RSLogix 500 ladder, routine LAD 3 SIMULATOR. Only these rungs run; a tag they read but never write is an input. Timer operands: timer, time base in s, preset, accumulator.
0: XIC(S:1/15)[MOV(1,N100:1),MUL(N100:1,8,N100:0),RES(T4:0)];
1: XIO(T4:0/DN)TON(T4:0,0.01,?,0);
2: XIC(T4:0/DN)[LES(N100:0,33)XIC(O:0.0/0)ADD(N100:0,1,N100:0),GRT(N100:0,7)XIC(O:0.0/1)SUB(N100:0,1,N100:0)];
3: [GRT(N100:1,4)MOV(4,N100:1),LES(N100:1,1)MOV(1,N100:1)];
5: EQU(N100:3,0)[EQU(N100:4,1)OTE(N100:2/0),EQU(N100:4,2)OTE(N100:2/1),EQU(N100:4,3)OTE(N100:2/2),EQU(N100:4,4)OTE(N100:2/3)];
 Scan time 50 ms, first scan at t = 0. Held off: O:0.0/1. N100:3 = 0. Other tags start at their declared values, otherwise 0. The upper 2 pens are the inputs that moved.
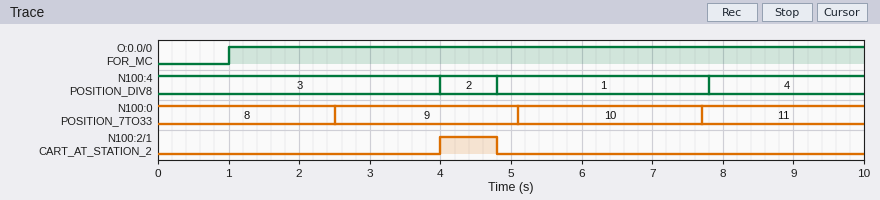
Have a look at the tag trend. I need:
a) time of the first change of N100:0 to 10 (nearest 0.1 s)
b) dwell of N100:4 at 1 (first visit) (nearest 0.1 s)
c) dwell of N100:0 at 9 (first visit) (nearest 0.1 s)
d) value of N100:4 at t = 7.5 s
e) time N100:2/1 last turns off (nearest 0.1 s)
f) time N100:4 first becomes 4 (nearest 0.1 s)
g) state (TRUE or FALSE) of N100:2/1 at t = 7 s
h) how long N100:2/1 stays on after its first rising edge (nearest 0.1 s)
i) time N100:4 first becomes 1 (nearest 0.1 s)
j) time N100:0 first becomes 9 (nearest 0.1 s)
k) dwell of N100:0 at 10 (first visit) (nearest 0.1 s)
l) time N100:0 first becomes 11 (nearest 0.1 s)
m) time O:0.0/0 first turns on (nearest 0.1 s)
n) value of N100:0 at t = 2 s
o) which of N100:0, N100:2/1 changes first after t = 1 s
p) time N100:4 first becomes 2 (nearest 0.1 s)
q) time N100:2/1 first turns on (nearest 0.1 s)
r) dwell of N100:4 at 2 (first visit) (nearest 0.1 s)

5.1 s
3.0 s
2.6 s
1
4.8 s
7.8 s
FALSE
0.8 s
4.8 s
2.5 s
2.6 s
7.7 s
1.0 s
8
N100:0
4.0 s
4.0 s
0.8 s
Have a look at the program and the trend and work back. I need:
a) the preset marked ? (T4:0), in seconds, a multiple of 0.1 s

2.5 s
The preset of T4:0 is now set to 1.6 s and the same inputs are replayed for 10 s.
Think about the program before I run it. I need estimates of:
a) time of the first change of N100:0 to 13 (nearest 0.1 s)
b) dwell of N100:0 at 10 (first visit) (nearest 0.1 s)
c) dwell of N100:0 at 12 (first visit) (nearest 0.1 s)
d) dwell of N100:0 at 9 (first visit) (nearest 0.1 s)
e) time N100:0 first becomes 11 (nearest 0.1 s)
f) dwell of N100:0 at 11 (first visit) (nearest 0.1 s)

8.4 s
1.7 s
1.7 s
1.7 s
5.0 s
1.7 s
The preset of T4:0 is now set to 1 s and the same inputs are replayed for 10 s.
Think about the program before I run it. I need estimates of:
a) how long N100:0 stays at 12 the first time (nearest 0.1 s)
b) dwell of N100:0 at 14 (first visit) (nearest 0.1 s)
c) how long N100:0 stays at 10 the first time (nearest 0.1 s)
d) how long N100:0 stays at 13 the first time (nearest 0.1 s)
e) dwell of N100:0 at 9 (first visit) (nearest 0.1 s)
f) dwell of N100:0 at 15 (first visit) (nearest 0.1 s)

1.1 s
1.1 s
1.1 s
1.1 s
1.1 s
1.1 s
